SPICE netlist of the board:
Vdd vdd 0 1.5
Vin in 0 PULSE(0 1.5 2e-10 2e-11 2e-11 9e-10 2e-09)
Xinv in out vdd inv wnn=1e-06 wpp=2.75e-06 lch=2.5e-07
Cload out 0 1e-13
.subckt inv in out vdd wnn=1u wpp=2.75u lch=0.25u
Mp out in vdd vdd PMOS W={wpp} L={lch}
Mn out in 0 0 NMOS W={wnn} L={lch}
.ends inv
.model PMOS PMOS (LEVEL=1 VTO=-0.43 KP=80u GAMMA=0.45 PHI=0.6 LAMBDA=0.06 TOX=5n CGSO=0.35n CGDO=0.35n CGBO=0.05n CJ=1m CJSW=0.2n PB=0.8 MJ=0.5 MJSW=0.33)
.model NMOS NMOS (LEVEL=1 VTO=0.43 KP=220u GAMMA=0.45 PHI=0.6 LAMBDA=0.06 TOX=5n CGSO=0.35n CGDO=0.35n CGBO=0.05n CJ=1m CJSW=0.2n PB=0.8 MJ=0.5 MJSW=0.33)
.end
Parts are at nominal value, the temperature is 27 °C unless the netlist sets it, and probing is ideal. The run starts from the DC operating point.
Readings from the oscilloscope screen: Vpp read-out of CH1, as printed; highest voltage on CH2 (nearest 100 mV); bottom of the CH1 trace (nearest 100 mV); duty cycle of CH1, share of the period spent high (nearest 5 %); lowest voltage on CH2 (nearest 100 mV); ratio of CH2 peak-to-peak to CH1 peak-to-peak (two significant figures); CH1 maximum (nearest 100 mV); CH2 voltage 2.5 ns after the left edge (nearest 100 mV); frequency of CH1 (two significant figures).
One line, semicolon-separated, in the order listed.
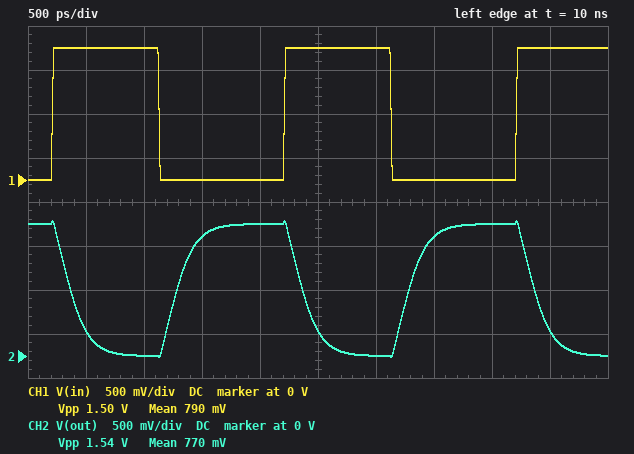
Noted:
1.50 V; 1.5 V; 0 V; 45 %; 0 V; 1.0; 1.5 V; 300 mV; 500 MHz
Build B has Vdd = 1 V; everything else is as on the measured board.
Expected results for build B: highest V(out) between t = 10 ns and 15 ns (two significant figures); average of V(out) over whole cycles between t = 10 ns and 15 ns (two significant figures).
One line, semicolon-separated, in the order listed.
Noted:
1.0 V; 410 mV
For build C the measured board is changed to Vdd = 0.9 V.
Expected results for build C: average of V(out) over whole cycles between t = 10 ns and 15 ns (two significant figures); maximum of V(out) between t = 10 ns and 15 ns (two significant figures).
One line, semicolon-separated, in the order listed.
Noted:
310 mV; 840 mV
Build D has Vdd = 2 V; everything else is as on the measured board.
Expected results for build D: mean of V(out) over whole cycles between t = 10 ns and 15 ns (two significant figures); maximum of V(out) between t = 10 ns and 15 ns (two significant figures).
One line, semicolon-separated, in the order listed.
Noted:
1.2 V; 2.0 V
